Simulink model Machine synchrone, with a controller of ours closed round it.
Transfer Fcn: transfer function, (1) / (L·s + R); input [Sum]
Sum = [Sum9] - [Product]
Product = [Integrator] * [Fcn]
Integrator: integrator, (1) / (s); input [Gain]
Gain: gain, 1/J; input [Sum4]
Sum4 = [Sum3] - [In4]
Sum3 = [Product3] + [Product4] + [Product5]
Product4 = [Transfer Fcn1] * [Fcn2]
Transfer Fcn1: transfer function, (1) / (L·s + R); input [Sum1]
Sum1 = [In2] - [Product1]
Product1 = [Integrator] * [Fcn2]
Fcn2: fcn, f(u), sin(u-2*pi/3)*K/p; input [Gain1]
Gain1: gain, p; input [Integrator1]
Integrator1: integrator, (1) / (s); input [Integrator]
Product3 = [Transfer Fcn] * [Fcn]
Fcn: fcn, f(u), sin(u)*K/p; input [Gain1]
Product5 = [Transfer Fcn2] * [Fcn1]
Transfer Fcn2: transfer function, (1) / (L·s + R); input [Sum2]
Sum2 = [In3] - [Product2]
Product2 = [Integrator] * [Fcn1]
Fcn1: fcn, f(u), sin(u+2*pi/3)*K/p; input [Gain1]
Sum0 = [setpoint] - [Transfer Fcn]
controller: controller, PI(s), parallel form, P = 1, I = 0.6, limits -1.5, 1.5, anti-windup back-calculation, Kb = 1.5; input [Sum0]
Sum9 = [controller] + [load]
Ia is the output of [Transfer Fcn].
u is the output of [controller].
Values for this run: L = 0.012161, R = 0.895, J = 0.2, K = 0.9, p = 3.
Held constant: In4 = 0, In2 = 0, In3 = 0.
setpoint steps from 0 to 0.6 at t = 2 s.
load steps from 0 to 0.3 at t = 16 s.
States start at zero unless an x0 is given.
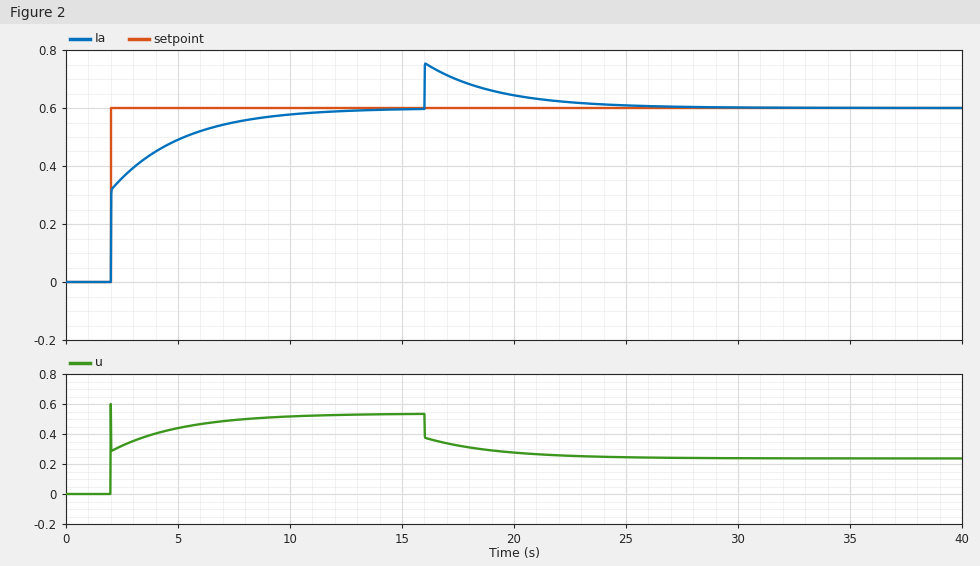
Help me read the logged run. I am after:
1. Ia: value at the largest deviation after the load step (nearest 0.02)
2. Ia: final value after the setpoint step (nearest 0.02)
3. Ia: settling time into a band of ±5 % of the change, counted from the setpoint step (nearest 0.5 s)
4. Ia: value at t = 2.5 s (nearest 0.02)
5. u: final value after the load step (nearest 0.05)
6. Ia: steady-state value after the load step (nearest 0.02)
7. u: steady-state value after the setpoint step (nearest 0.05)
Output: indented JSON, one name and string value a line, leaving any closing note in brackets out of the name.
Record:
{
  "Ia: value at the largest deviation after the load step": "0.76",
  "Ia: final value after the setpoint step": "0.60",
  "Ia: settling time into a band of ±5 % of the change, counted from the setpoint step": "7.0 s",
  "Ia: value at t = 2.5 s": "0.36",
  "u: final value after the load step": "0.25",
  "Ia: steady-state value after the load step": "0.60",
  "u: steady-state value after the setpoint step": "0.55"
}
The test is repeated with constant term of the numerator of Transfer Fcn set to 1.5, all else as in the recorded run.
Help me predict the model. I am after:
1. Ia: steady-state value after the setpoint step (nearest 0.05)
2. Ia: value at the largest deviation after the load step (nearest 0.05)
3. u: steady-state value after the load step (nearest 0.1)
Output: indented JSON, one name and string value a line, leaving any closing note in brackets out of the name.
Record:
{
  "Ia: steady-state value after the setpoint step": "0.60",
  "Ia: value at the largest deviation after the load step": "0.80",
  "u: steady-state value after the load step": "0.1"
}
